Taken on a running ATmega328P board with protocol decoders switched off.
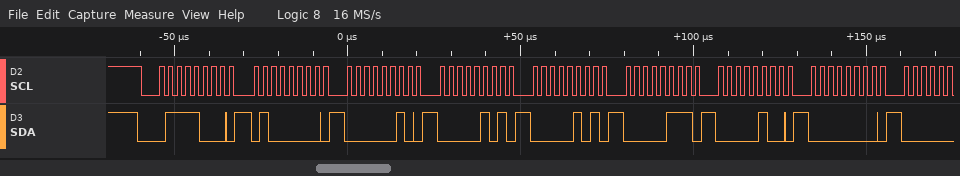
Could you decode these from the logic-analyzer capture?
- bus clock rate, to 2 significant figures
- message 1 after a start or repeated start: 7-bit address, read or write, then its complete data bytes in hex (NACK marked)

400 kHz
0x3C write: 40 02 05 05 07 04 00
